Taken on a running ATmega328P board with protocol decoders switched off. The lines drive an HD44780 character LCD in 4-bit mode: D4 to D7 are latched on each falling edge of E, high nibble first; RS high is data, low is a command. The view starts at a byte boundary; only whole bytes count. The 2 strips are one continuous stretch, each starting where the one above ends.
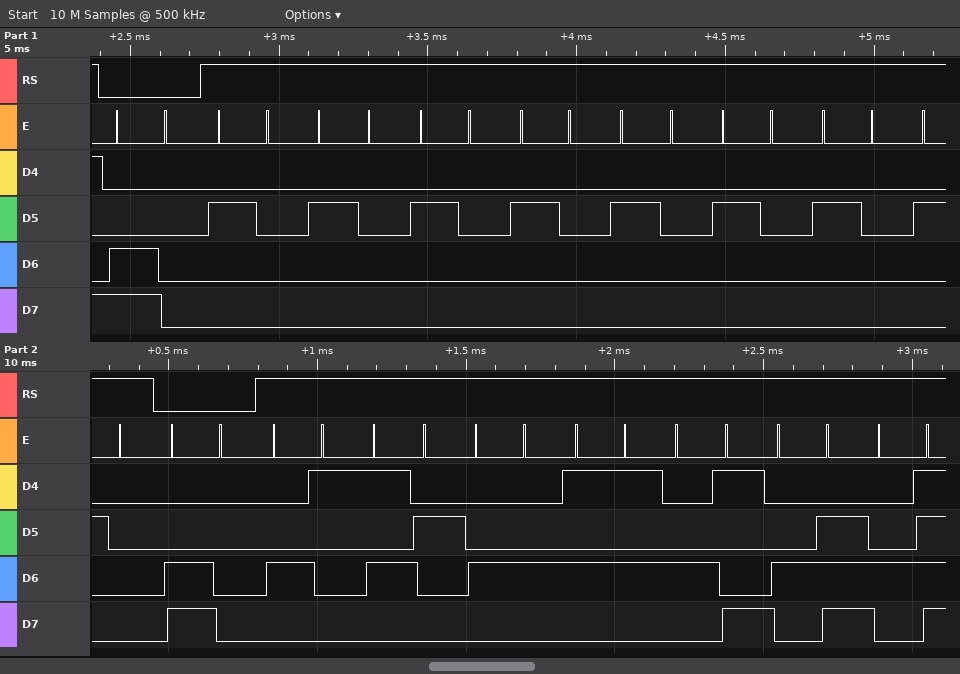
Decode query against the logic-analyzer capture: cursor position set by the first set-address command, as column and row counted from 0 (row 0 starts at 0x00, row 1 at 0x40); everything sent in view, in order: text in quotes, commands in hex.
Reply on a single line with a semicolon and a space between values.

column 0, row 1; 0xC0 "        " 0xC0 "ARDUINO"
